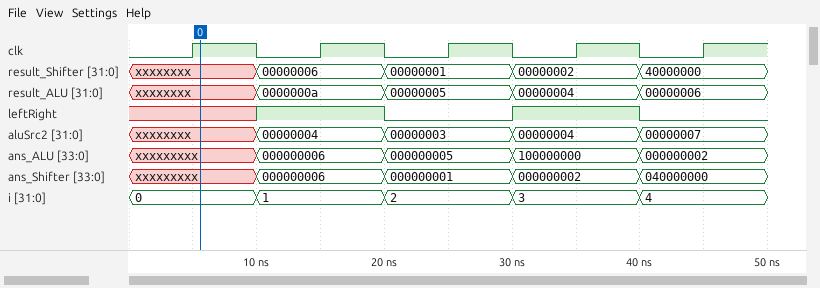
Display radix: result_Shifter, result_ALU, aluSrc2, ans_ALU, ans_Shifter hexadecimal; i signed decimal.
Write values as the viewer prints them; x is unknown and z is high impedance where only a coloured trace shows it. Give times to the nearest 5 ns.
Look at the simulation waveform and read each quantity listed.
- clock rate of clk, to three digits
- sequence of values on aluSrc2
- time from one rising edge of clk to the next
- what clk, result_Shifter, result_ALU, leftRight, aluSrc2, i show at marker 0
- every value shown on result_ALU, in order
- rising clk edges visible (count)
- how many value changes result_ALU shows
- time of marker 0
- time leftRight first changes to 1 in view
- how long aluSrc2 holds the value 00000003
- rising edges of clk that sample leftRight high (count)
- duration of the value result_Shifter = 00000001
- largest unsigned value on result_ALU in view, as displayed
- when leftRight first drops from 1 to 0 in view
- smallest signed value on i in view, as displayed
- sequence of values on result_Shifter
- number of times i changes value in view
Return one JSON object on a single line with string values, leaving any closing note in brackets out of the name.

{"clock rate of clk, to three digits": "100 MHz", "sequence of values on aluSrc2": "xxxxxxxx, 00000004, 00000003, 00000004, 00000007", "time from one rising edge of clk to the next": "10 ns", "what clk, result_Shifter, result_ALU, leftRight, aluSrc2, i show at marker 0": "clk=1, result_Shifter=xxxxxxxx, result_ALU=xxxxxxxx, leftRight=x, aluSrc2=xxxxxxxx, i=0", "every value shown on result_ALU, in order": "xxxxxxxx, 0000000a, 00000005, 00000004, 00000006", "rising clk edges visible": "5", "how many value changes result_ALU shows": "4", "time of marker 0": "5 ns", "time leftRight first changes to 1 in view": "10 ns", "how long aluSrc2 holds the value 00000003": "10 ns", "rising edges of clk that sample leftRight high": "2", "duration of the value result_Shifter = 00000001": "10 ns", "largest unsigned value on result_ALU in view, as displayed": "0000000a", "when leftRight first drops from 1 to 0 in view": "20 ns", "smallest signed value on i in view, as displayed": "0", "sequence of values on result_Shifter": "xxxxxxxx, 00000006, 00000001, 00000002, 40000000", "number of times i changes value in view": "4"}
